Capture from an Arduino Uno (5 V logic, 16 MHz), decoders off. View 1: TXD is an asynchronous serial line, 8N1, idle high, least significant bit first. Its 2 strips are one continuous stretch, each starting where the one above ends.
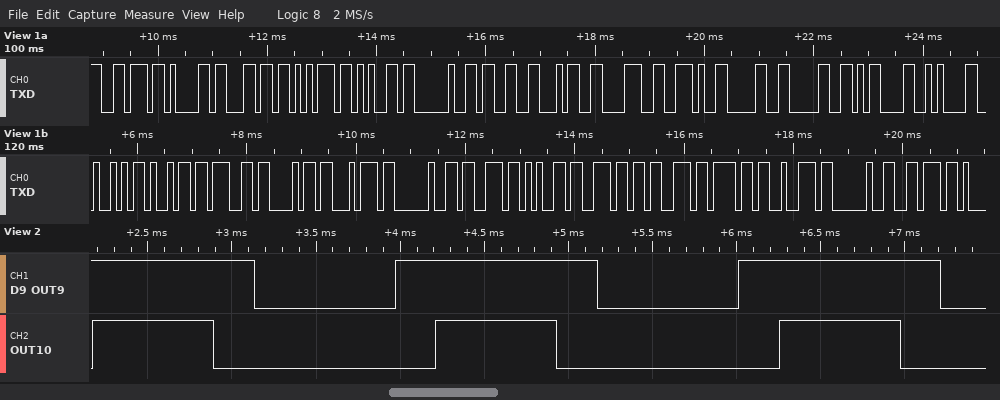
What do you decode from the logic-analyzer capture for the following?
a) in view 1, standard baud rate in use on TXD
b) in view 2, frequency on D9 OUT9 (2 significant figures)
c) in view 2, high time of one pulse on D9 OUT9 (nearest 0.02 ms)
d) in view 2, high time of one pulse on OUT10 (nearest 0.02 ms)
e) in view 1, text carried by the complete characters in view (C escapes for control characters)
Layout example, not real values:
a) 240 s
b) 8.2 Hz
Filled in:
a) 9600 baud
b) 490 Hz
c) 1.20 ms
d) 0.72 ms
e) "value 348.00\r\nRight sensor v"
